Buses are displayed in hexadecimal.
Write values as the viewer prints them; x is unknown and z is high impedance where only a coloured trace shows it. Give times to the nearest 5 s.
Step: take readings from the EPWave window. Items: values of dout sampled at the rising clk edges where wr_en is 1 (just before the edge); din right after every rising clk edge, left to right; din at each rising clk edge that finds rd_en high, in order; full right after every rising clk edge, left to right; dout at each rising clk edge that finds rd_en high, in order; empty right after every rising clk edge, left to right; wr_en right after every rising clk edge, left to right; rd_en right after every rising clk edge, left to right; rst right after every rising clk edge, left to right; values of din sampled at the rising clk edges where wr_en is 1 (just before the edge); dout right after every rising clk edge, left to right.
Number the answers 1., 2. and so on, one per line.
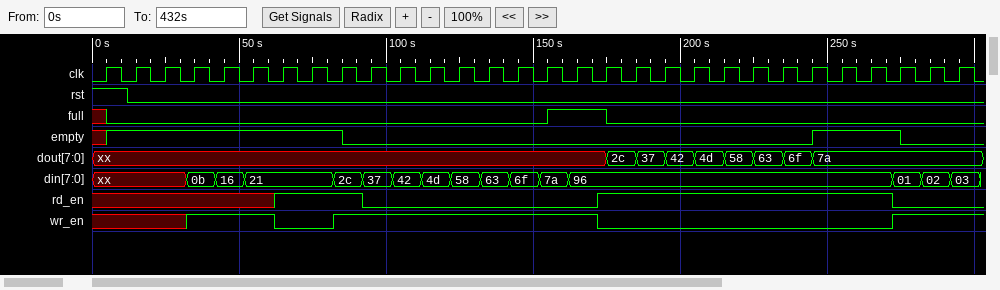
1. xx, xx, xx, xx, xx, xx, xx, xx, xx, xx, xx, xx, 7a, 7a, 7a
2. xx, xx, xx, 0b, 16, 21, 21, 21, 2c, 37, 42, 4d, 58, 63, 6f, 7a, 96, 96, 96, 96, 96, 96, 96, 96, 96, 96, 96, 01, 02, 03
3. 21, 21, 2c, 96, 96, 96, 96, 96, 96, 96, 96, 96, 96
4. 0 0 0 0 0 0 0 0 0 0 0 0 0 0 0 1 1 0 0 0 0 0 0 0 0 0 0 0 0 0
5. xx, xx, xx, xx, 2c, 37, 42, 4d, 58, 63, 6f, 7a, 7a
6. 1 1 1 1 1 1 1 1 0 0 0 0 0 0 0 0 0 0 0 0 0 0 0 0 1 1 1 0 0 0
7. x x x 1 1 1 0 0 1 1 1 1 1 1 1 1 1 0 0 0 0 0 0 0 0 0 0 1 1 1
8. x x x x x x 1 1 1 0 0 0 0 0 0 0 0 1 1 1 1 1 1 1 1 1 1 0 0 0
9. 1 0 0 0 0 0 0 0 0 0 0 0 0 0 0 0 0 0 0 0 0 0 0 0 0 0 0 0 0 0
10. 0b, 16, 21, 2c, 37, 42, 4d, 58, 63, 6f, 7a, 96, 01, 02, 03
11. xx, xx, xx, xx, xx, xx, xx, xx, xx, xx, xx, xx, xx, xx, xx, xx, xx, 2c, 37, 42, 4d, 58, 63, 6f, 7a, 7a, 7a, 7a, 7a, 7a
